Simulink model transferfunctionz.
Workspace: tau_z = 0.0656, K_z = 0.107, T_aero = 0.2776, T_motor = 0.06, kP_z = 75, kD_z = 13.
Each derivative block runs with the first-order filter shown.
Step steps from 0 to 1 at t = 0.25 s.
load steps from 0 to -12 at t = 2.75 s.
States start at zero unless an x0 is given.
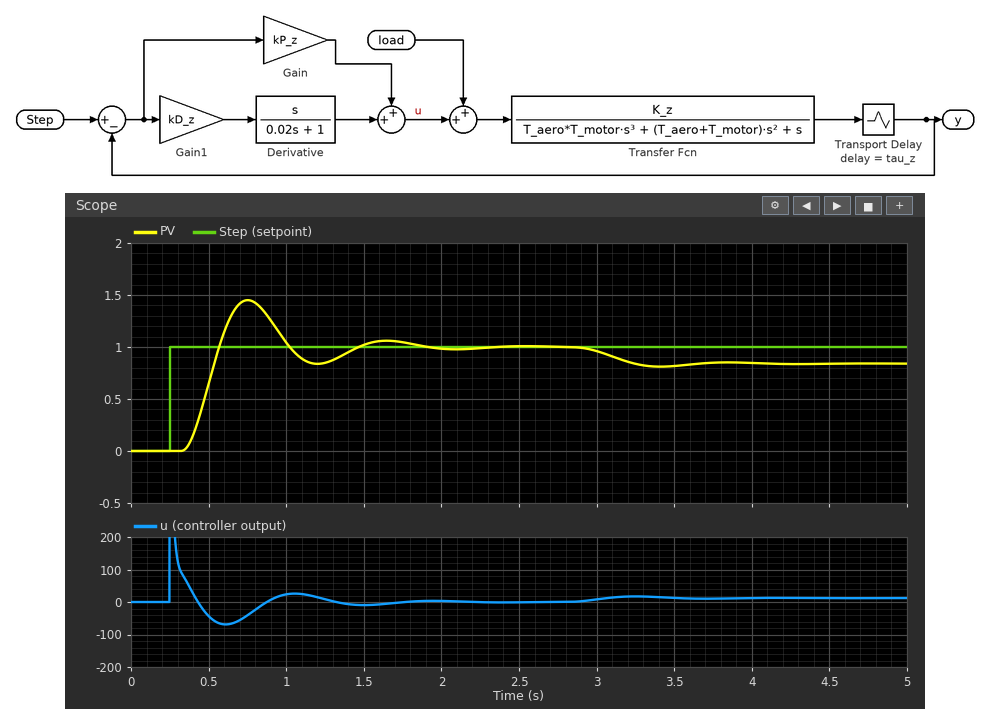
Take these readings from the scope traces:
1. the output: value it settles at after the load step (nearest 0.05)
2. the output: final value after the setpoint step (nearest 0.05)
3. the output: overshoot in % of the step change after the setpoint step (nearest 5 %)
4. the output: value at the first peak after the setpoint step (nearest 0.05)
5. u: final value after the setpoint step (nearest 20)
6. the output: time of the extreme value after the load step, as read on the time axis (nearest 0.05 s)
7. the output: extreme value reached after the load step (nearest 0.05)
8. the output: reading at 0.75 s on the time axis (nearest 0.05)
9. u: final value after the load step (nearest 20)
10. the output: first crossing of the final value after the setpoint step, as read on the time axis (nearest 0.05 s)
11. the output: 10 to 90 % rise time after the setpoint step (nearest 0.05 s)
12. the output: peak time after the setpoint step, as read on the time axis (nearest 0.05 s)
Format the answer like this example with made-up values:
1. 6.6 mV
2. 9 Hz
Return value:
1. 0.85
2. 1.00
3. 45 %
4. 1.45
5. 0
6. 3.40 s
7. 0.80
8. 1.45
9. 20
10. 0.55 s
11. 0.15 s
12. 0.75 s
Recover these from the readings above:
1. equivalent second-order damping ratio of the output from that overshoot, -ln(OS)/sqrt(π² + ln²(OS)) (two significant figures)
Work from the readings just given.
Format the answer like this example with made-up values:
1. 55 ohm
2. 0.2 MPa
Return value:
1. 0.25
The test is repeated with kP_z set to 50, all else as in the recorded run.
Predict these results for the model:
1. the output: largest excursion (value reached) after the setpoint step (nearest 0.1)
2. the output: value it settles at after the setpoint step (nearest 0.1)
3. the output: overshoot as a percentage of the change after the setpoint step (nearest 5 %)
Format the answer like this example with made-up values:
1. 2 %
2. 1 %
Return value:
1. 1.2
2. 1.0
3. 20 %
